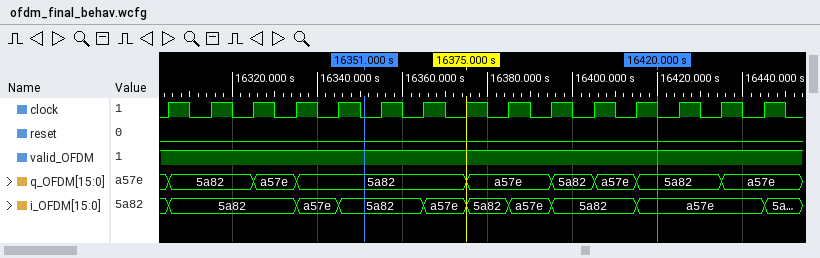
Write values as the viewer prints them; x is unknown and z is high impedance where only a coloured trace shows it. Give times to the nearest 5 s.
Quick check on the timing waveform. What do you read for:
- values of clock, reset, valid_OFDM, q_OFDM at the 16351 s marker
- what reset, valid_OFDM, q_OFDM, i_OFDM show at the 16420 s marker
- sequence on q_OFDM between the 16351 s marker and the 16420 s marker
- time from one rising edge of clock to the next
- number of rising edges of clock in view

clock=0, reset=0, valid_OFDM=1, q_OFDM=5a82
reset=0, valid_OFDM=1, q_OFDM=5a82, i_OFDM=a57e
5a82, a57e, 5a82, a57e, 5a82
10 s
15
